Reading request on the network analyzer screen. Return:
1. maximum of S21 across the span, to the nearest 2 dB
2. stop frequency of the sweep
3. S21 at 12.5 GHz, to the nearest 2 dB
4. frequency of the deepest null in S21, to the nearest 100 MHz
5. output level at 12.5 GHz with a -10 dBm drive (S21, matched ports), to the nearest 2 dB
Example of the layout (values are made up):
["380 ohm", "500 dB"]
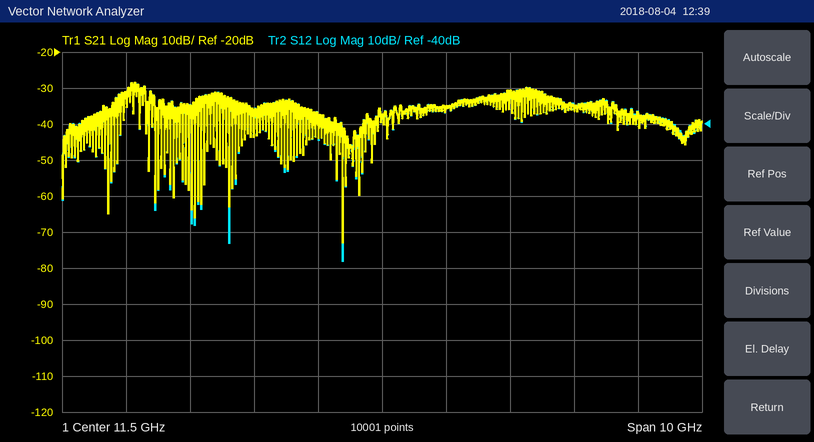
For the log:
["-28 dB", "16.5 GHz", "-36 dB", "10.9 GHz", "-46 dBm"]
